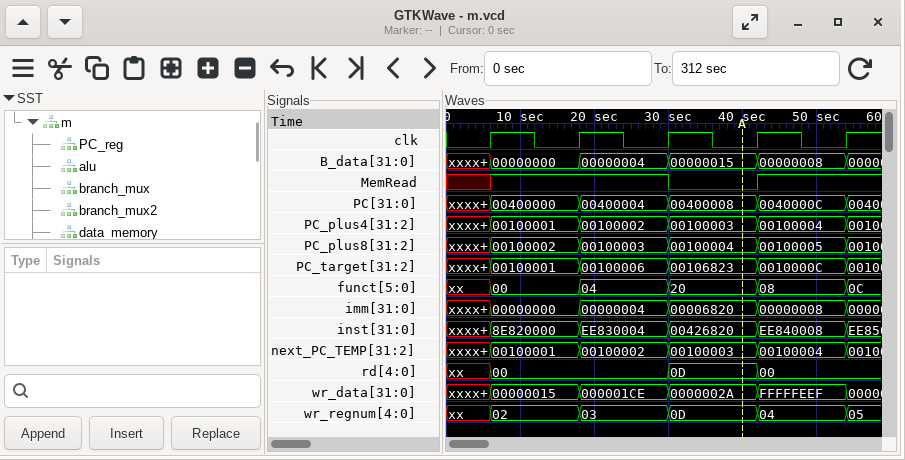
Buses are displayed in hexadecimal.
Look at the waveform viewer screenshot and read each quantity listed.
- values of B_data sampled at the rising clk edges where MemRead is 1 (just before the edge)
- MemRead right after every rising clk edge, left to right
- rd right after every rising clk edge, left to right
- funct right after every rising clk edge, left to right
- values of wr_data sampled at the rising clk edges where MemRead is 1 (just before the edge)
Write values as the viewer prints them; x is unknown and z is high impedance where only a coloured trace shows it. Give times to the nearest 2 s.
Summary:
00000000, 00000004, 00000008
1 1 0 1 1
00, 00, 0D, 00, 00
00, 04, 20, 08, 0C
00000015, 000001CE, FFFFFEEF
